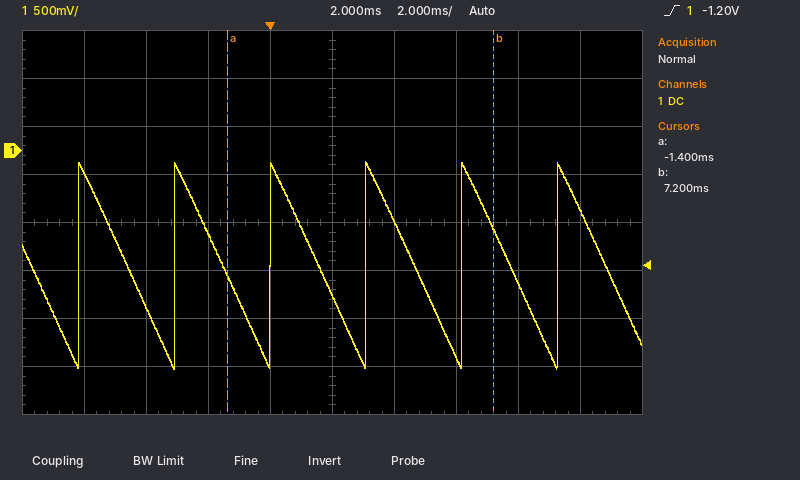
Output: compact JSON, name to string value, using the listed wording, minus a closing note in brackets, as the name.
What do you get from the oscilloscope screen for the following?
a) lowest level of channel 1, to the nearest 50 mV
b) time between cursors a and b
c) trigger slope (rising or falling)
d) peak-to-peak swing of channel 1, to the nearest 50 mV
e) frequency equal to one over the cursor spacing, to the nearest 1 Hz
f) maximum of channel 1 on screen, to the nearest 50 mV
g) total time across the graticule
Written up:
{"lowest level of channel 1, to the nearest 50 mV": "-2.25 V", "time between cursors a and b": "8.6 ms", "trigger slope": "rising", "peak-to-peak swing of channel 1, to the nearest 50 mV": "2.15 V", "frequency equal to one over the cursor spacing, to the nearest 1 Hz": "116 Hz", "maximum of channel 1 on screen, to the nearest 50 mV": "-100 mV", "total time across the graticule": "20 ms"}
